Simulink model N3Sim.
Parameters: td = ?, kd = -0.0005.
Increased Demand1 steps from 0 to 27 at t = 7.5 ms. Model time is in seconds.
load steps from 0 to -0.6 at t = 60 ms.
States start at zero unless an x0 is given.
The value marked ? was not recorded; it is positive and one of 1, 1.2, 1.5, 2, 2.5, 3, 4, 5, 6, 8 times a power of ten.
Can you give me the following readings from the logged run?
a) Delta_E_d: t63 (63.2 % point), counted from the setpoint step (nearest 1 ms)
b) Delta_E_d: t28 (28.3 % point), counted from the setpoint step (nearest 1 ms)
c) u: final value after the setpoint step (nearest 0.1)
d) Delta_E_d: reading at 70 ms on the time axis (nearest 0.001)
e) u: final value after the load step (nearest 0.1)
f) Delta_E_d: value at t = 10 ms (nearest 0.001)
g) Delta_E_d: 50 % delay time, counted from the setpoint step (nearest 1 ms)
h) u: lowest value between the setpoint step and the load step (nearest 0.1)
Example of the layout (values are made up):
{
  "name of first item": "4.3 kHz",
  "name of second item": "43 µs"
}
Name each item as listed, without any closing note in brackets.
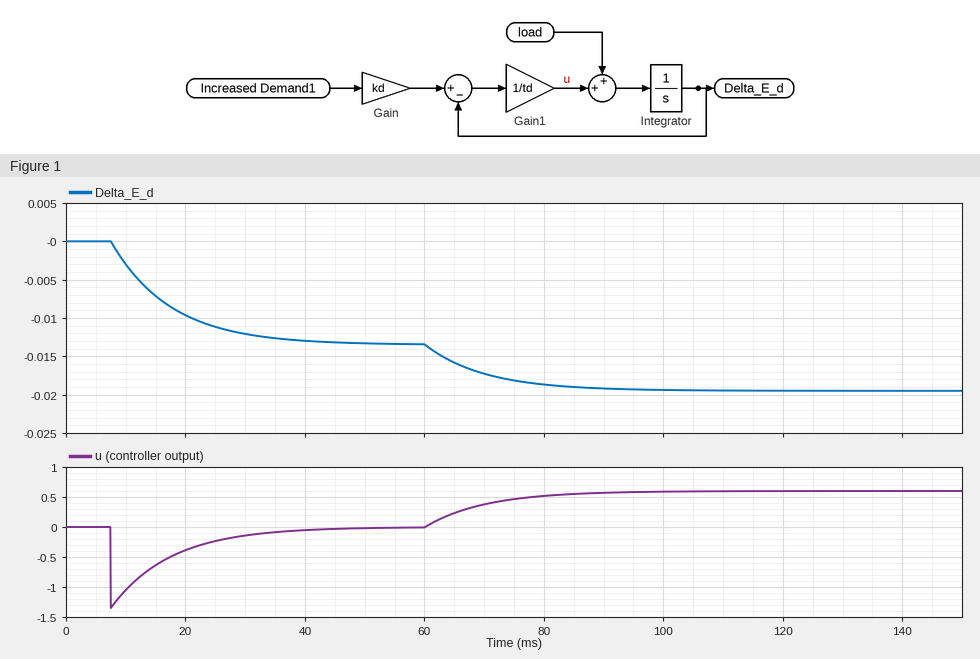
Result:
{
  "Delta_E_d: t63 (63.2 % point), counted from the setpoint step": "10 ms",
  "Delta_E_d: t28 (28.3 % point), counted from the setpoint step": "3 ms",
  "u: final value after the setpoint step": "0.0",
  "Delta_E_d: reading at 70 ms on the time axis": "-0.017",
  "u: final value after the load step": "0.6",
  "Delta_E_d: value at t = 10 ms": "-0.003",
  "Delta_E_d: 50 % delay time, counted from the setpoint step": "7 ms",
  "u: lowest value between the setpoint step and the load step": "-1.3"
}
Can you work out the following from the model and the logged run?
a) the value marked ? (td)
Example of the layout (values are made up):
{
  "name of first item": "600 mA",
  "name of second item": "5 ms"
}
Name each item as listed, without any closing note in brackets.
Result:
{
  "the value marked ?": "0.01"
}
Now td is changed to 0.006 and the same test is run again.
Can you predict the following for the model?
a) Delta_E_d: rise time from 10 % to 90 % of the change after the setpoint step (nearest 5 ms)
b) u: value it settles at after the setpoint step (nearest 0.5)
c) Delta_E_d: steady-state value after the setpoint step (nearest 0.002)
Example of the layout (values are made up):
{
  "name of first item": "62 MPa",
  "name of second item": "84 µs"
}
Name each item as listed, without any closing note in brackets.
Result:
{
  "Delta_E_d: rise time from 10 % to 90 % of the change after the setpoint step": "15 ms",
  "u: value it settles at after the setpoint step": "0.0",
  "Delta_E_d: steady-state value after the setpoint step": "-0.014"
}
